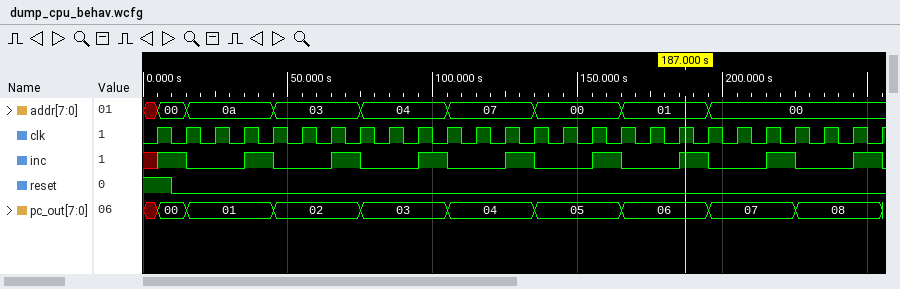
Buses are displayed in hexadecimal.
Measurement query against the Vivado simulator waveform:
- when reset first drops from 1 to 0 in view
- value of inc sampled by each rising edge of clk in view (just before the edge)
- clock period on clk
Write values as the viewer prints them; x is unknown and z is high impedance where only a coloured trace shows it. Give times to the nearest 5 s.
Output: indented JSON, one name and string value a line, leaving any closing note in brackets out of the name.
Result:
{
  "when reset first drops from 1 to 0 in view": "10 s",
  "value of inc sampled by each rising edge of clk in view": "x 1 0 0 1 0 0 1 0 0 1 0 0 1 0 0 1 0 0 1 0 0 1 0 0 1",
  "clock period on clk": "10 s"
}
